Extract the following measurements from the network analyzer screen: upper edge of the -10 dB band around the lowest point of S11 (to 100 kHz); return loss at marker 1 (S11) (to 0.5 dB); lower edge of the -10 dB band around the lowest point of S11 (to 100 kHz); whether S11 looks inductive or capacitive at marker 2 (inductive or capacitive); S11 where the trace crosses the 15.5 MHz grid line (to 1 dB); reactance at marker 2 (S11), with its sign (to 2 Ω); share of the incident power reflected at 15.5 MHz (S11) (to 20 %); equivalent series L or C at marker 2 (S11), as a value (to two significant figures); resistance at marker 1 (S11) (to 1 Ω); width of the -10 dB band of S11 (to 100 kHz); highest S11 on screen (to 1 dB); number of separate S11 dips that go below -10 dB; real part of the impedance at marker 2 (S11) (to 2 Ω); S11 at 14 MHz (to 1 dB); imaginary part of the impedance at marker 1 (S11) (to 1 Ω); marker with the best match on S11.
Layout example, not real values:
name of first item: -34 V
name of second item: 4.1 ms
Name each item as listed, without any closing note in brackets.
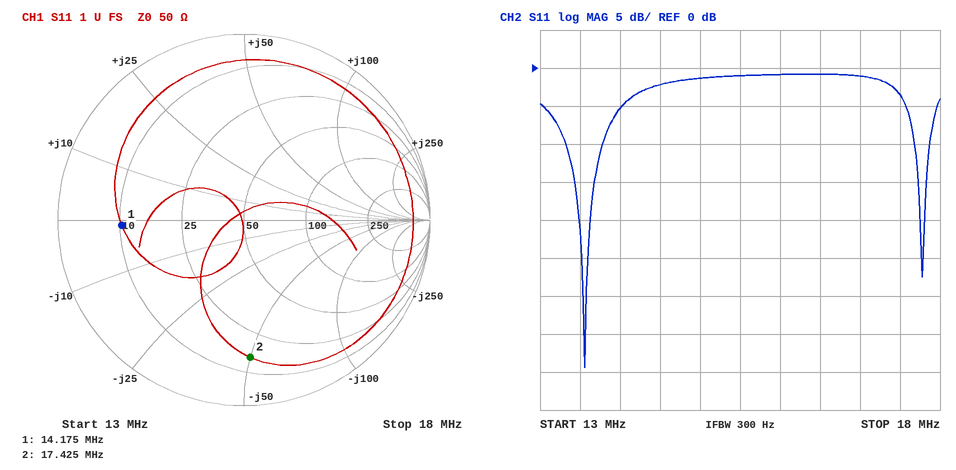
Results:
upper edge of the -10 dB band around the lowest point of S11: 13.8 MHz
return loss at marker 1 (S11): 3.5 dB
lower edge of the -10 dB band around the lowest point of S11: 13.3 MHz
whether S11 looks inductive or capacitive at marker 2: capacitive
S11 where the trace crosses the 15.5 MHz grid line: -1 dB
reactance at marker 2 (S11), with its sign: -50 Ω
share of the incident power reflected at 15.5 MHz (S11): 80 %
equivalent series L or C at marker 2 (S11), as a value: 180 pF
resistance at marker 1 (S11): 10 Ω
width of the -10 dB band of S11: 500 kHz
highest S11 on screen: -1 dB
number of separate S11 dips that go below -10 dB: 2
real part of the impedance at marker 2 (S11): 16 Ω
S11 at 14 MHz: -5 dB
imaginary part of the impedance at marker 1 (S11): -1 Ω
marker with the best match on S11: marker 1
